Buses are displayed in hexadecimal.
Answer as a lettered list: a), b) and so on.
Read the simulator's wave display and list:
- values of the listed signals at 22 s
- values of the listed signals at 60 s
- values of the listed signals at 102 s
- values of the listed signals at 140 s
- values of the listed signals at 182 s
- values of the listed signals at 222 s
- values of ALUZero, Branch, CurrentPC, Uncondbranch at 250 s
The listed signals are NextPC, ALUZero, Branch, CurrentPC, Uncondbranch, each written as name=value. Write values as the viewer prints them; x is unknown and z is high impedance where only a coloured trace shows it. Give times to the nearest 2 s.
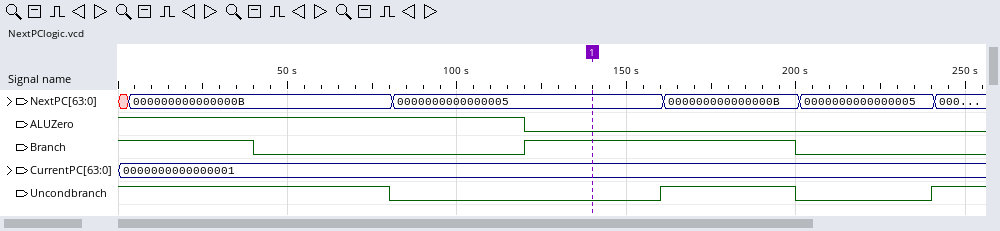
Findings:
a) NextPC=000000000000000B, ALUZero=1, Branch=1, CurrentPC=0000000000000001, Uncondbranch=1
b) NextPC=000000000000000B, ALUZero=1, Branch=0, CurrentPC=0000000000000001, Uncondbranch=1
c) NextPC=0000000000000005, ALUZero=1, Branch=0, CurrentPC=0000000000000001, Uncondbranch=0
d) NextPC=0000000000000005, ALUZero=0, Branch=1, CurrentPC=0000000000000001, Uncondbranch=0
e) NextPC=000000000000000B, ALUZero=0, Branch=1, CurrentPC=0000000000000001, Uncondbranch=1
f) NextPC=0000000000000005, ALUZero=0, Branch=0, CurrentPC=0000000000000001, Uncondbranch=0
g) ALUZero=0, Branch=0, CurrentPC=0000000000000001, Uncondbranch=1
